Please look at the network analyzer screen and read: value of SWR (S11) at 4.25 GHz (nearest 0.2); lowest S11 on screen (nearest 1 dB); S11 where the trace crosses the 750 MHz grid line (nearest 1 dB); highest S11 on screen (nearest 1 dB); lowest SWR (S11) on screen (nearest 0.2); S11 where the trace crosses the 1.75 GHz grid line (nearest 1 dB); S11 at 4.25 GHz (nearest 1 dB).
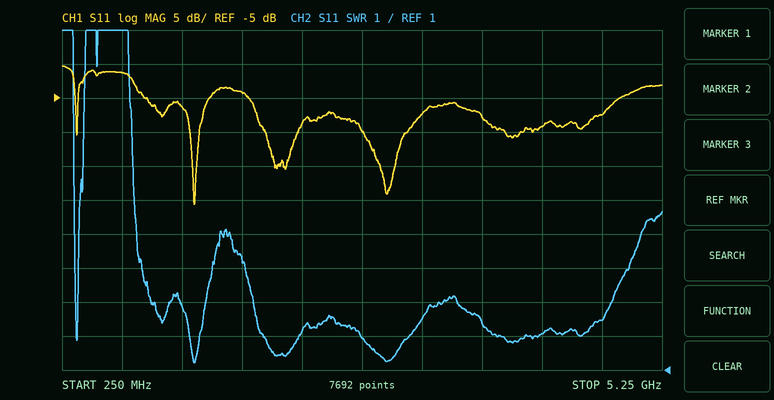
2.0
-21 dB
-1 dB
0 dB
1.2
-4 dB
-9 dB
